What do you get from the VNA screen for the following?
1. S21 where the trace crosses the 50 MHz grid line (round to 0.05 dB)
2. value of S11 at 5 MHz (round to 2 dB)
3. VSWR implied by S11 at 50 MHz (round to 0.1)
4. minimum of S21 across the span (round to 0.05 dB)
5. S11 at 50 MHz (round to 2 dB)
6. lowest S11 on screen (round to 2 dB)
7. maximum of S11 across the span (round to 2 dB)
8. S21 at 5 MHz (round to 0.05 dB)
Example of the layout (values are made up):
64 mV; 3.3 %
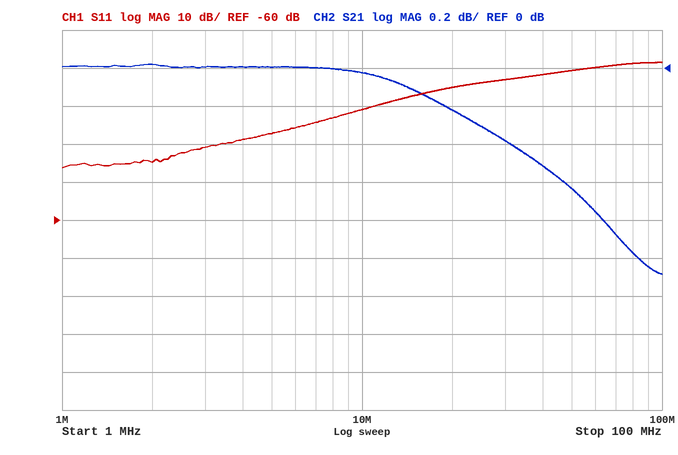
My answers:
-0.65 dB; -38 dB; 1.2; -1.10 dB; -20 dB; -46 dB; -18 dB; 0.00 dB
